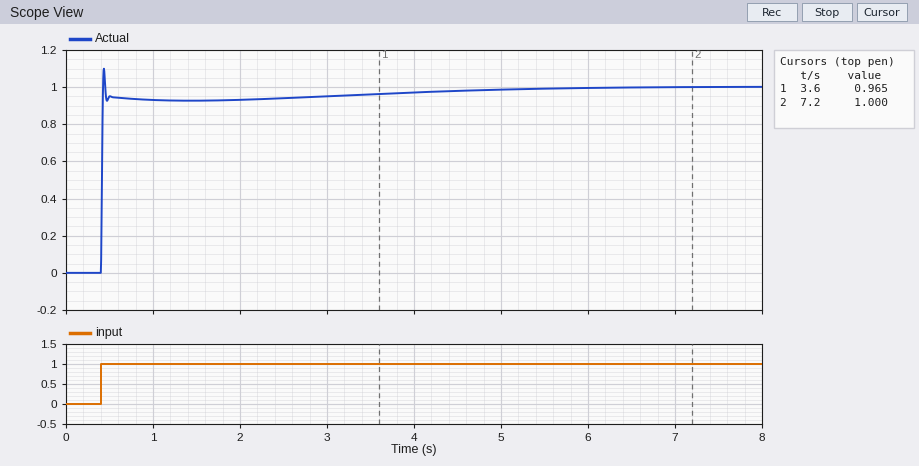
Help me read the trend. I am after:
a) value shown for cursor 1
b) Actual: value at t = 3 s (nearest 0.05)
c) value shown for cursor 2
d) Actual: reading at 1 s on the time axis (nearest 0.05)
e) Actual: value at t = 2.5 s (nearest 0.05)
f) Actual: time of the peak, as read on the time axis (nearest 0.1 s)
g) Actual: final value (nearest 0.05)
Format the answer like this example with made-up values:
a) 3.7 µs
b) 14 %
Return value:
a) 0.965
b) 0.95
c) 1.000
d) 0.95
e) 0.95
f) 0.4 s
g) 1.00
